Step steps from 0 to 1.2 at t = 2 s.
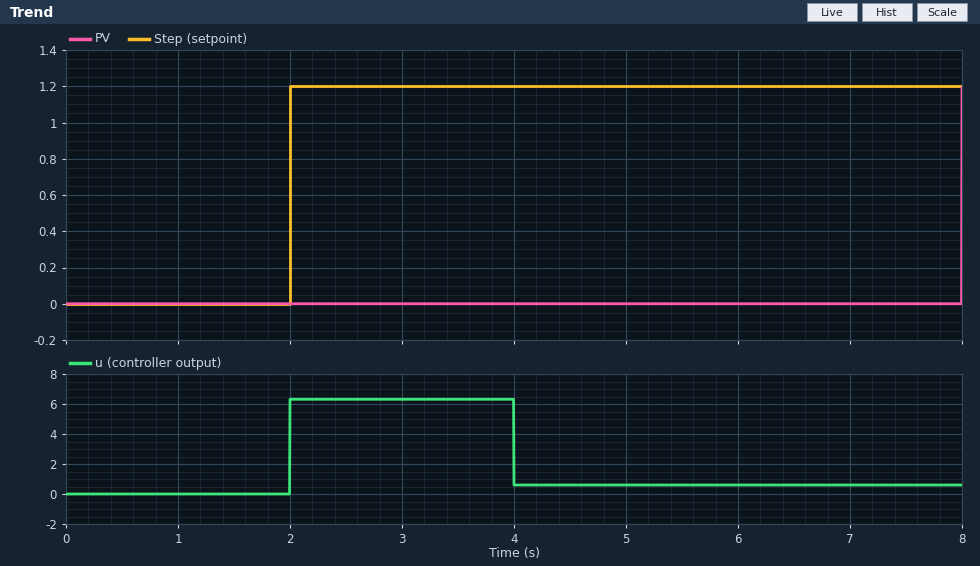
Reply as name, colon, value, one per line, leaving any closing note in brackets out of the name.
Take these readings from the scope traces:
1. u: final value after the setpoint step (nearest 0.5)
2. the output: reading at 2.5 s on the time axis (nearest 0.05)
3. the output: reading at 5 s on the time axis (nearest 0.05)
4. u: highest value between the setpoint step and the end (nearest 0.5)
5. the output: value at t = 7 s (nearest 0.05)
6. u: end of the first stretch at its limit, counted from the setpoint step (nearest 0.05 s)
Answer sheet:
u: final value after the setpoint step: 0.5
the output: reading at 2.5 s on the time axis: 0.00
the output: reading at 5 s on the time axis: 0.00
u: highest value between the setpoint step and the end: 6.5
the output: value at t = 7 s: 0.00
u: end of the first stretch at its limit, counted from the setpoint step: 2.00 s
